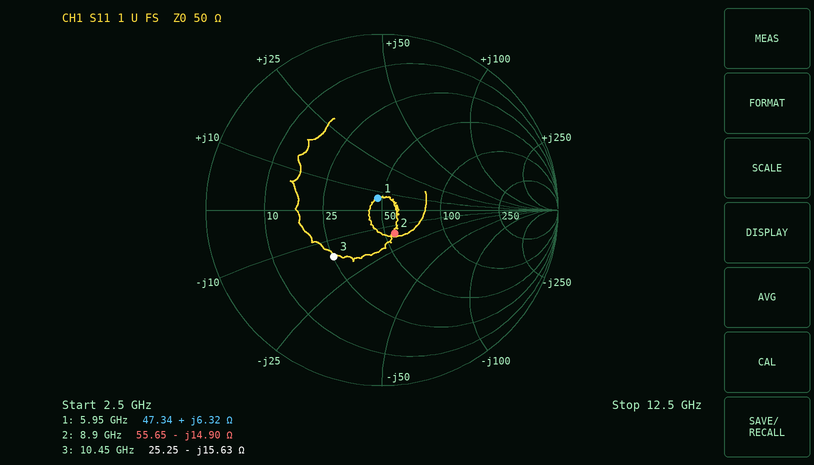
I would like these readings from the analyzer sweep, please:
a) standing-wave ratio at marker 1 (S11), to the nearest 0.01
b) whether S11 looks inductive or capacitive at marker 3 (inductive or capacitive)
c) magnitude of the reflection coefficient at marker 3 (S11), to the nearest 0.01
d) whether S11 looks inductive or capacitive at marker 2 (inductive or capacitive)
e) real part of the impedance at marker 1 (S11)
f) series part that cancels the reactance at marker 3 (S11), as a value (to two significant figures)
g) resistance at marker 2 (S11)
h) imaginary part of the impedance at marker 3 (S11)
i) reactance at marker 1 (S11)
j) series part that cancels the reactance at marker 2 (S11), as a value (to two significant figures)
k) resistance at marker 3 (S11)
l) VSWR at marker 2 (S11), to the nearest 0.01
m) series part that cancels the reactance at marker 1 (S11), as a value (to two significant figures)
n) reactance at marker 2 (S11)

1.15
capacitive
0.38
capacitive
47.34 Ω
240 pH
55.65 Ω
-15.63 Ω
+6.32 Ω
270 pH
25.25 Ω
1.35
4.2 pF
-14.90 Ω
